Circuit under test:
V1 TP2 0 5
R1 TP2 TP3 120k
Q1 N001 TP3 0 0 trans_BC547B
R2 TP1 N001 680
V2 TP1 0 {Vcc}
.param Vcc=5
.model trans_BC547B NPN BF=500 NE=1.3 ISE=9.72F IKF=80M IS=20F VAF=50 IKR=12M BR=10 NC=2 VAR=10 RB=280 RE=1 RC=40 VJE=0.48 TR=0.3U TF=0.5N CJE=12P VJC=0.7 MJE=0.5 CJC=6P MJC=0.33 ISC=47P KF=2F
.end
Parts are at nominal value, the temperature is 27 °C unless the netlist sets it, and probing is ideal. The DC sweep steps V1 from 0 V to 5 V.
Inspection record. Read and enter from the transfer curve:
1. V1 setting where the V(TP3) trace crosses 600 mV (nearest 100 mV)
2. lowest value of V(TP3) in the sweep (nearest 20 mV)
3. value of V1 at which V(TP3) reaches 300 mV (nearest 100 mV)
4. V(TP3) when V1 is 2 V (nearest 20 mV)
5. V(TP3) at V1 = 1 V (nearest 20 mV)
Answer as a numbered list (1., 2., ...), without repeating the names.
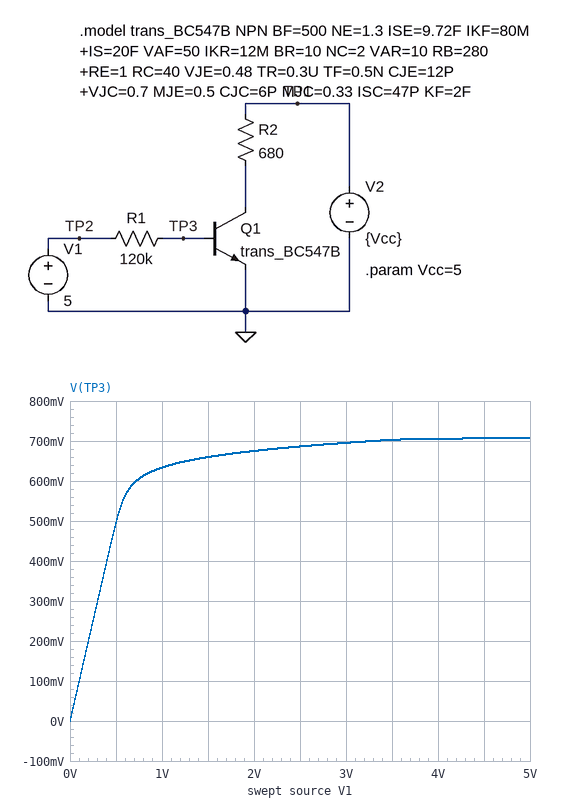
1. 700 mV
2. 0 V
3. 300 mV
4. 680 mV
5. 640 mV
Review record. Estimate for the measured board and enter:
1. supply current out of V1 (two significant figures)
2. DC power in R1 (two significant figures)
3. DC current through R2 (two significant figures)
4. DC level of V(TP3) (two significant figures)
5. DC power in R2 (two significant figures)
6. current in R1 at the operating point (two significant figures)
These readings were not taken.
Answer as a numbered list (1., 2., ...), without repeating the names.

1. 36 µA
2. 150 µW
3. 6.8 mA
4. 710 mV
5. 31 mW
6. 36 µA
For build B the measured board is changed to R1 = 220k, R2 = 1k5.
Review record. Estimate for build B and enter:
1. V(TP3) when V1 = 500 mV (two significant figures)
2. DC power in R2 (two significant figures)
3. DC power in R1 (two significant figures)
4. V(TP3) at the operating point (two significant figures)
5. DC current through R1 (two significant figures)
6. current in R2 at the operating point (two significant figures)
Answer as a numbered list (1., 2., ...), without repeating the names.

1. 490 mV
2. 15 mW
3. 85 µW
4. 680 mV
5. 20 µA
6. 3.2 mA
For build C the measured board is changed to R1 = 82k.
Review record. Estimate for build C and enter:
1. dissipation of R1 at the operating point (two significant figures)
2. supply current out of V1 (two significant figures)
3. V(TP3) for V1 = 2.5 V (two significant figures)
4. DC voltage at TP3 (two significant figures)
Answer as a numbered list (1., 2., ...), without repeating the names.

1. 220 µW
2. 52 µA
3. 700 mV
4. 710 mV
